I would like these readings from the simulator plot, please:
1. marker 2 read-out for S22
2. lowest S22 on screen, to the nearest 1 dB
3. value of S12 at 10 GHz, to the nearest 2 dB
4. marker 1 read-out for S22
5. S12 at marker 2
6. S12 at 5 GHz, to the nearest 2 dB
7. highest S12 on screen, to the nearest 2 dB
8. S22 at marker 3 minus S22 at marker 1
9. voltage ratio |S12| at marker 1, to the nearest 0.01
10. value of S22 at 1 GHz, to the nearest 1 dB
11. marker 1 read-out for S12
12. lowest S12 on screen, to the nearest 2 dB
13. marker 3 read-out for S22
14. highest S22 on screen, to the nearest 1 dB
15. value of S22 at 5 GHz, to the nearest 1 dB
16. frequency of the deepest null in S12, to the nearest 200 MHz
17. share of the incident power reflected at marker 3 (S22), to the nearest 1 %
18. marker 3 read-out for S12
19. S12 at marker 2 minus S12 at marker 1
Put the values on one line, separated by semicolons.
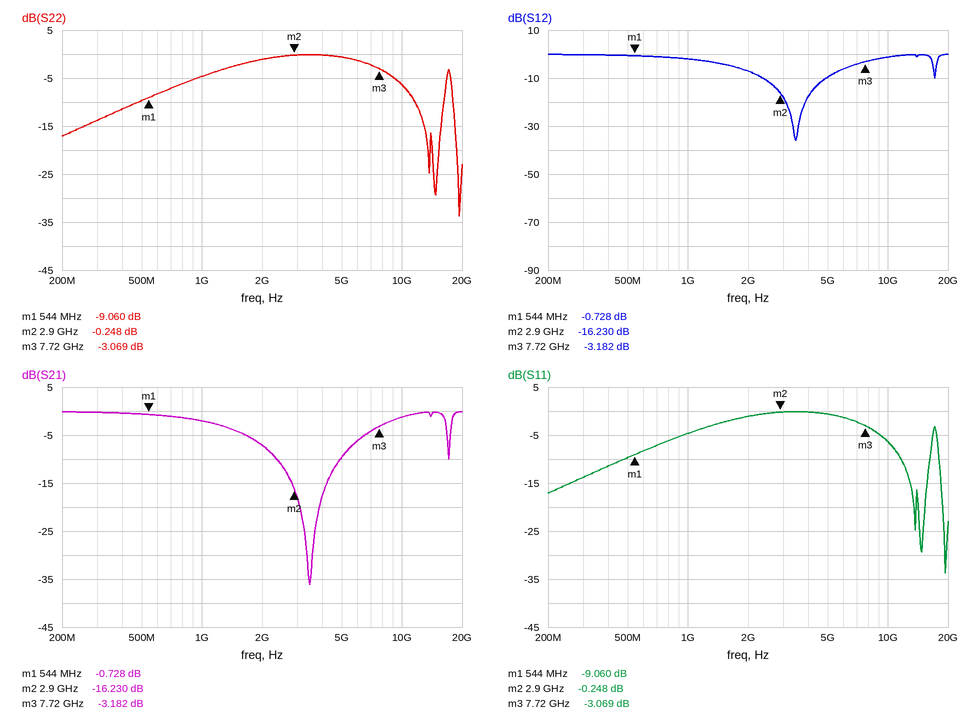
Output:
-0.248 dB; -34 dB; -2 dB; -9.060 dB; -16.230 dB; -10 dB; 0 dB; 5.991 dB; 0.92; -5 dB; -0.728 dB; -36 dB; -3.069 dB; 0 dB; -1 dB; 3.4 GHz; 49 %; -3.182 dB; -15.502 dB
